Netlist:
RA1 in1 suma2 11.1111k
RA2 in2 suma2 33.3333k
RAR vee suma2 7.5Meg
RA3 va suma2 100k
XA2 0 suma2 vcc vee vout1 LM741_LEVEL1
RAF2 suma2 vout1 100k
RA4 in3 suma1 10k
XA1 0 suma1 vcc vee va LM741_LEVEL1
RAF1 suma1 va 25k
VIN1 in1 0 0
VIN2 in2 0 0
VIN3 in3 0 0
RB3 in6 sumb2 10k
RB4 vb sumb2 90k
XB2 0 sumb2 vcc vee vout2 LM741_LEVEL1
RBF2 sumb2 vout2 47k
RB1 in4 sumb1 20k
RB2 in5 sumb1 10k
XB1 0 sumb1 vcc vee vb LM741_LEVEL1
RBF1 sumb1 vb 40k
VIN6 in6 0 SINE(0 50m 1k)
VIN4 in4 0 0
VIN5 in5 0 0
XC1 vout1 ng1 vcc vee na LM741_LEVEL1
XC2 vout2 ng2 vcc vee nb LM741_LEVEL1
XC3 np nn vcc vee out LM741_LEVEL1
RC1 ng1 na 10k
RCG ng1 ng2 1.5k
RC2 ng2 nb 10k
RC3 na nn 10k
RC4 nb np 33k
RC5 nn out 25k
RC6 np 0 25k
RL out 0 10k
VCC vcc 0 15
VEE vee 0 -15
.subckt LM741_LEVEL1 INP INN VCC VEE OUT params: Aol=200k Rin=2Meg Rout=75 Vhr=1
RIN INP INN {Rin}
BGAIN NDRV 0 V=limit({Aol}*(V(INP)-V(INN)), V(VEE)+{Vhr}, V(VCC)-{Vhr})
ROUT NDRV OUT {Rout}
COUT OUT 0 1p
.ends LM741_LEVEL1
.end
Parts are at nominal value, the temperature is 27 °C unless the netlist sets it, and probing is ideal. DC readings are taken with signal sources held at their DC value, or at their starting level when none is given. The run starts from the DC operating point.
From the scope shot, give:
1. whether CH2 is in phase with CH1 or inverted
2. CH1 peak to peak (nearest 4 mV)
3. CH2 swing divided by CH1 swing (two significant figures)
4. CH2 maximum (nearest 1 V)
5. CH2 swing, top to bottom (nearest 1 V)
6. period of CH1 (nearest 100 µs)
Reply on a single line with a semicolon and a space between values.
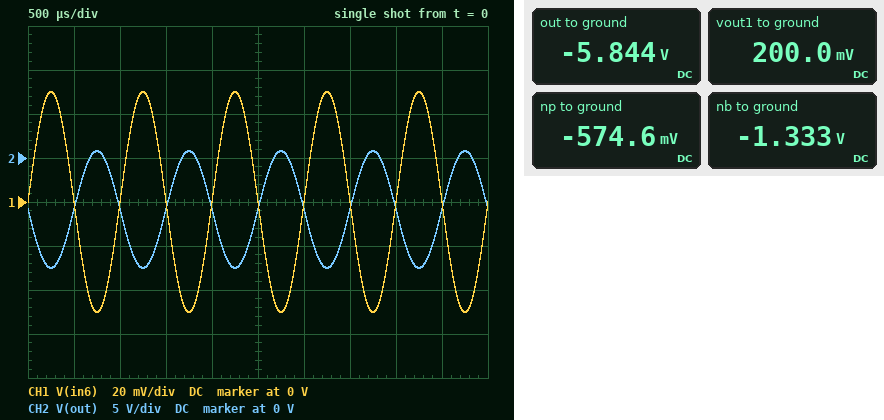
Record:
inverted; 100 mV; 130; 1 V; 13 V; 1.0 ms
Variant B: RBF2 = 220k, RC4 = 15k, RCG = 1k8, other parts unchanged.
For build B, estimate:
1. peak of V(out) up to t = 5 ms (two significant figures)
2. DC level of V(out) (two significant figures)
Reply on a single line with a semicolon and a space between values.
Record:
14 V; -5.7 V
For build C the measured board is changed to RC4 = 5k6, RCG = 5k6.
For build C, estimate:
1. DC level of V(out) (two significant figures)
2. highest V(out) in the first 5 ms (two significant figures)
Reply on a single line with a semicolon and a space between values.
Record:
-2.4 V; 510 mV
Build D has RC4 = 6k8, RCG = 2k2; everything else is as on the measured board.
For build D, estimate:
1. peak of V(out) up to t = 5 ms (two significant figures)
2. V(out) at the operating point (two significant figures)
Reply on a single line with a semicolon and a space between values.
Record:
980 mV; -5.3 V
